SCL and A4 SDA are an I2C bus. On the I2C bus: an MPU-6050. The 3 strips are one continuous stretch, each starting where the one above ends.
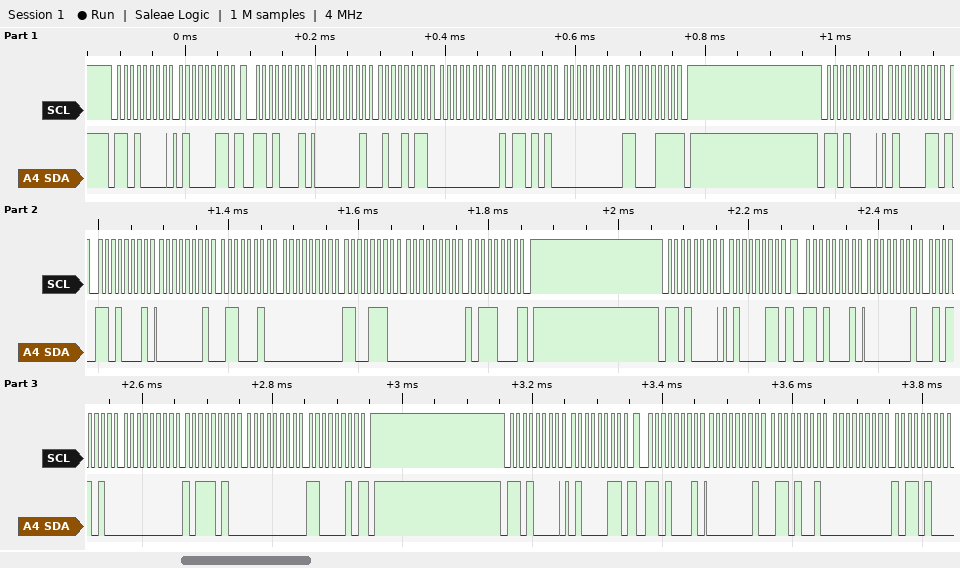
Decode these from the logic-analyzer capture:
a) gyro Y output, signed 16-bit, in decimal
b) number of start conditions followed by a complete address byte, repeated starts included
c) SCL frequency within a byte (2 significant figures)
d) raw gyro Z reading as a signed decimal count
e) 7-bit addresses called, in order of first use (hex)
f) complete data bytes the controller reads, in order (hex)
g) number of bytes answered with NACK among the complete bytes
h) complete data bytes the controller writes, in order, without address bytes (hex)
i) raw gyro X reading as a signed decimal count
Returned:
181
8
100 kHz
199
0x68
01 4B 00 B5 00 C7 01 62 00 CE 00 B8 01 5A 00 BA 00 C2 01 69 00 B4
3
43 43 43 43
331
